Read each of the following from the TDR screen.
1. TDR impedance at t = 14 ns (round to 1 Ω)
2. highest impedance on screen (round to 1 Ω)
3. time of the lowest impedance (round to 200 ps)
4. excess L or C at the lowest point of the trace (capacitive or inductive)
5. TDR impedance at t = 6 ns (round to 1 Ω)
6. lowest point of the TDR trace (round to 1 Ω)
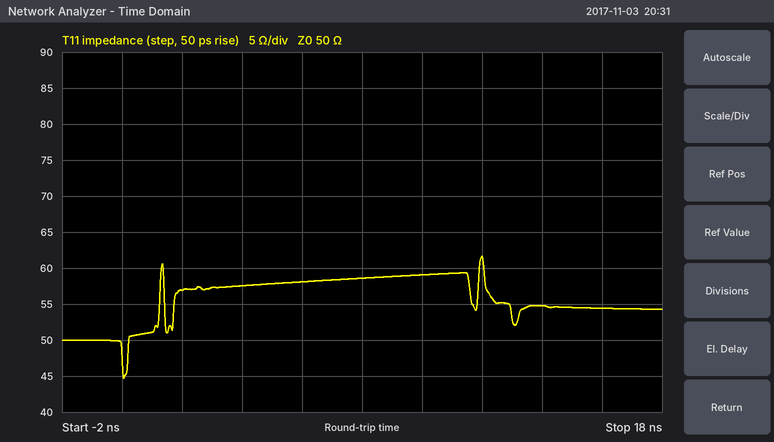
55 Ω
62 Ω
0.0 ns
capacitive
58 Ω
45 Ω
